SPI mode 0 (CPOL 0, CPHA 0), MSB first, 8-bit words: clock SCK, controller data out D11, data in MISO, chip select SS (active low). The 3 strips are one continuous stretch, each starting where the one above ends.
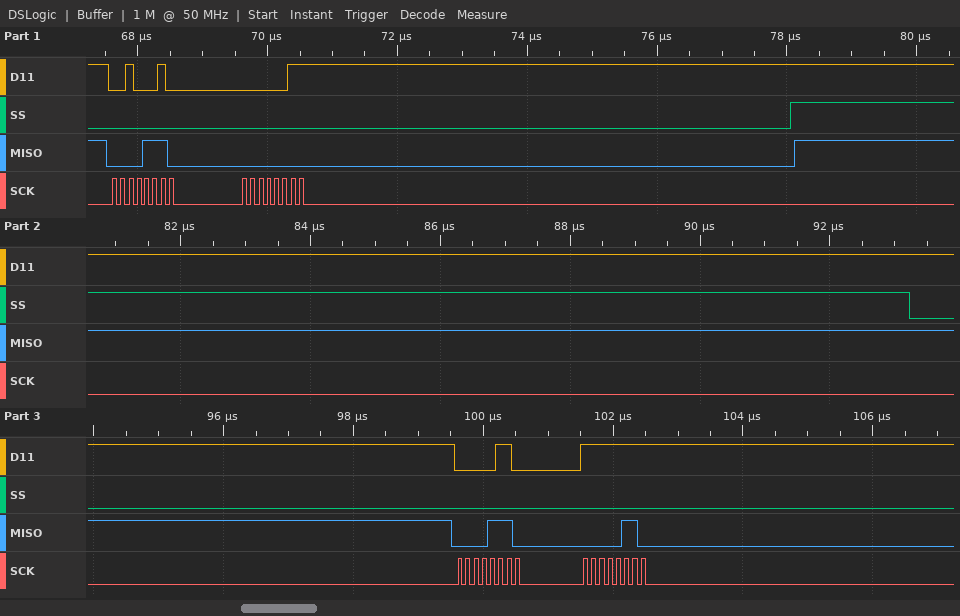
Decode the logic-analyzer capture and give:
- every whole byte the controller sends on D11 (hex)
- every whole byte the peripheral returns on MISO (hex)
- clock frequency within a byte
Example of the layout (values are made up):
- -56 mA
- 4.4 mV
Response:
- 22 03 06 FF
- 0E 00 0E 06
- 8 MHz
